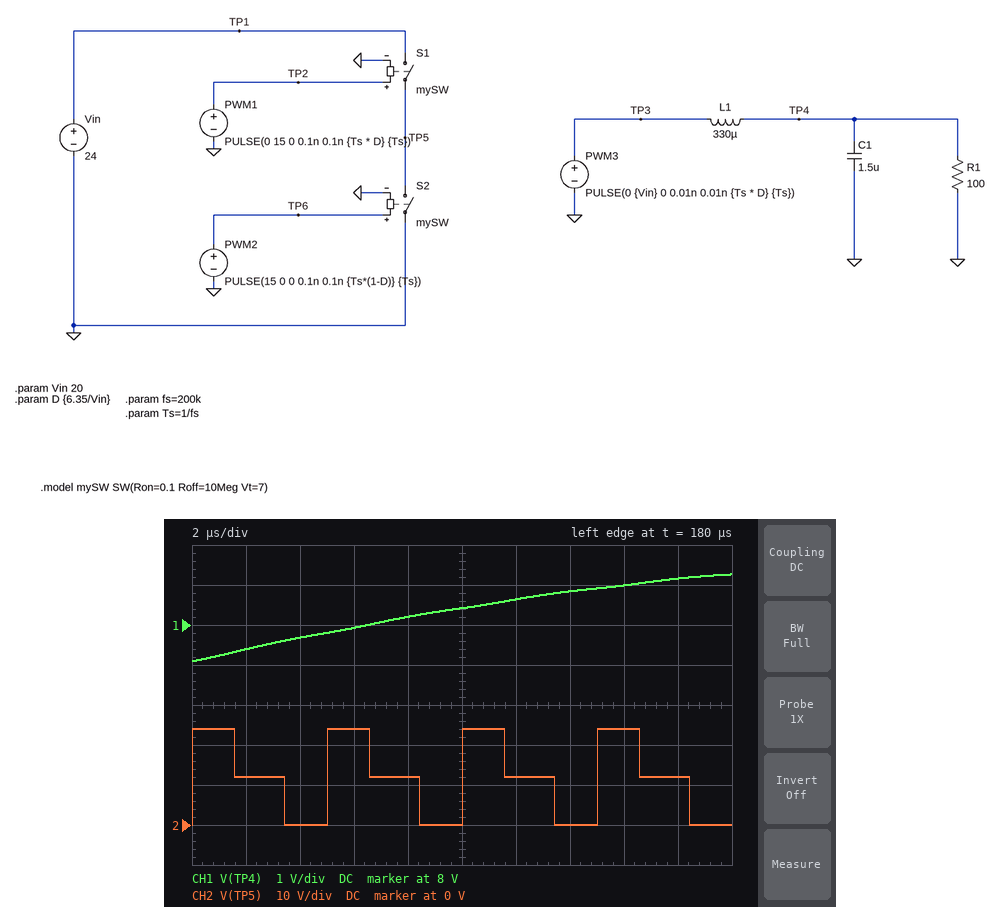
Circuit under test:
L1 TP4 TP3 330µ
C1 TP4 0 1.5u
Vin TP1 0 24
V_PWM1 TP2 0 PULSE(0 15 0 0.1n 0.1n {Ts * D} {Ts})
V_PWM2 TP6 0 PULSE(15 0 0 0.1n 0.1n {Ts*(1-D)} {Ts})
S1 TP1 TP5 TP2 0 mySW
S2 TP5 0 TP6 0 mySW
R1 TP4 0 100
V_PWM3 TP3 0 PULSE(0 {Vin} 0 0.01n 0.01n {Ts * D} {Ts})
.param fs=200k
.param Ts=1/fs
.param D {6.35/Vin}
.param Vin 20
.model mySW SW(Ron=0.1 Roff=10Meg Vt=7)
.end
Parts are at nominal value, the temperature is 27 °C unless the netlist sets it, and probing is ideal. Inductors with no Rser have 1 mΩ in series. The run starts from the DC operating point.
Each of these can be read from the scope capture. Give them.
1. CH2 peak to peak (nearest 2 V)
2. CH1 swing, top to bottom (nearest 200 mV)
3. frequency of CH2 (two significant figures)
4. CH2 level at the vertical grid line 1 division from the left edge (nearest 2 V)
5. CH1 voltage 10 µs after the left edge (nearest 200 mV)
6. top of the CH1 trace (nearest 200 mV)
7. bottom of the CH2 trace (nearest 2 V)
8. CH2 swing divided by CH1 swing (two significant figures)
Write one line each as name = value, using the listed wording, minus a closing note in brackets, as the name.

CH2 peak to peak = 24 V
CH1 swing, top to bottom = 2.2 V
frequency of CH2 = 200 kHz
CH2 level at the vertical grid line 1 division from the left edge = 12 V
CH1 voltage 10 µs after the left edge = 8.4 V
top of the CH1 trace = 9.2 V
bottom of the CH2 trace = 0 V
CH2 swing divided by CH1 swing = 11
